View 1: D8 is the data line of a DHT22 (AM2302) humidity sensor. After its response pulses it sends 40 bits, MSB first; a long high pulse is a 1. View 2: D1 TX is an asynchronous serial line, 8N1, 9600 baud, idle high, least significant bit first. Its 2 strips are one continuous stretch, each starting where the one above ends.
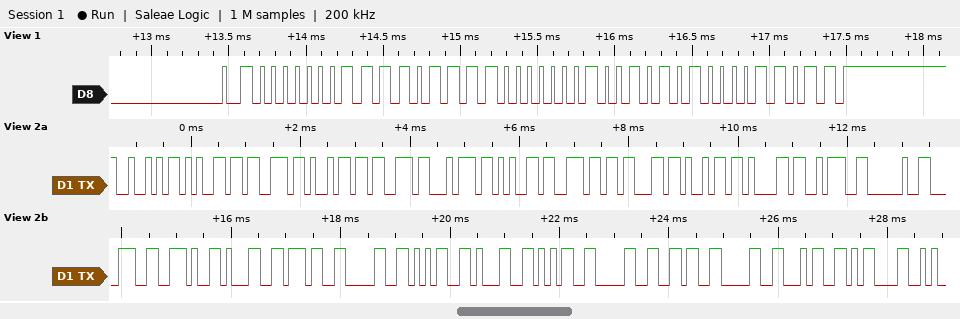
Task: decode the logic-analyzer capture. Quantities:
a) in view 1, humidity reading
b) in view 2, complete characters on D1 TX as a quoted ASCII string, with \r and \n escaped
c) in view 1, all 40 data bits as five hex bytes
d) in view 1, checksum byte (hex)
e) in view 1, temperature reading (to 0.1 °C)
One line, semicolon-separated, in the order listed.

49.5 %; "Resistencia: 8.1705150604\r"; 01 EF 01 2A 1B; 0x1B; 29.8 °C
